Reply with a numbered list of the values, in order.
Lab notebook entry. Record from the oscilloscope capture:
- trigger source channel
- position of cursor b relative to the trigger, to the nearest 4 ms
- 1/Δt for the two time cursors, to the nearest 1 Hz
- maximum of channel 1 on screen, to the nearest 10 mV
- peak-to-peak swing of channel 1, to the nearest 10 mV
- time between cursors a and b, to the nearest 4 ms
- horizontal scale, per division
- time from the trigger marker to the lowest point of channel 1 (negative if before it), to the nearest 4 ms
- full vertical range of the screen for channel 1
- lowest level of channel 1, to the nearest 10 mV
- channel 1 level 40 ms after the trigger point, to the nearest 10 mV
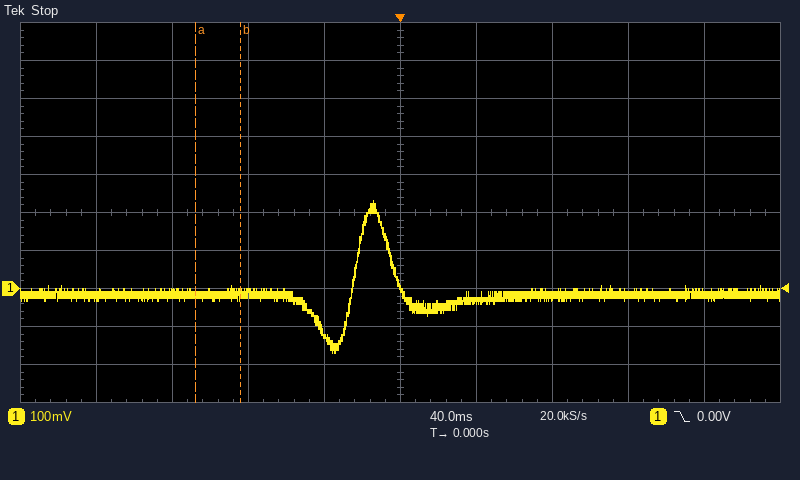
1. channel 1
2. -84 ms
3. 42 Hz
4. 230 mV
5. 400 mV
6. 24 ms
7. 40 ms
8. -36 ms
9. 1 V
10. -170 mV
11. -30 mV
